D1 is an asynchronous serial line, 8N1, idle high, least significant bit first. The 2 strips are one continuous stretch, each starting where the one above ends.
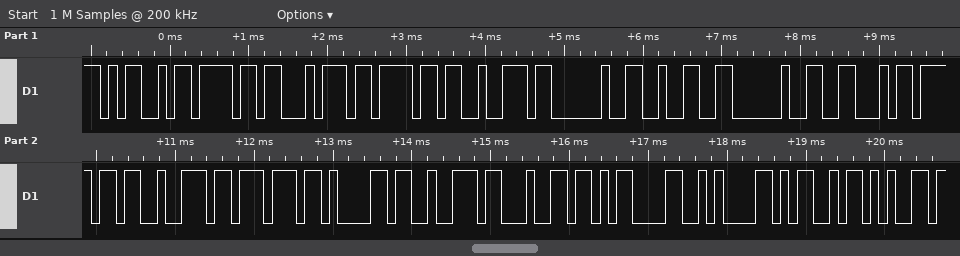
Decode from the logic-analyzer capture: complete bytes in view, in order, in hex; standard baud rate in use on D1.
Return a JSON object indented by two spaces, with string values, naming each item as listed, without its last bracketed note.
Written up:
{
  "complete bytes in view, in order, in hex": "0x4D 0x6F 0x74 0x6F 0x72 0x20 0x32 0x20 0x46 0x6F 0x72 0x77 0x61 0x72 0x64 0x0D 0x0A 0x4D 0x65",
  "standard baud rate in use on D1": "9600 baud"
}
